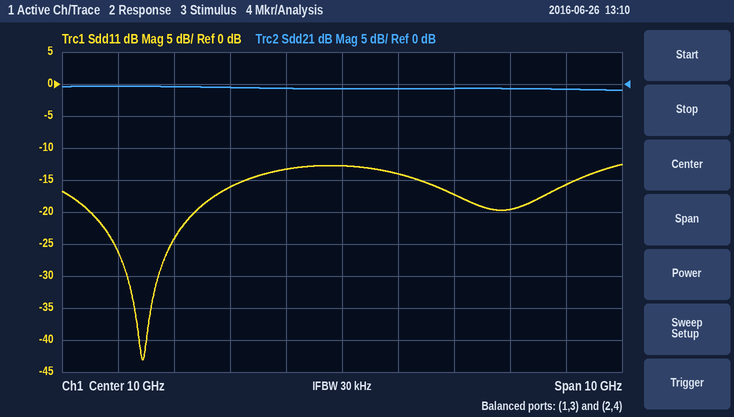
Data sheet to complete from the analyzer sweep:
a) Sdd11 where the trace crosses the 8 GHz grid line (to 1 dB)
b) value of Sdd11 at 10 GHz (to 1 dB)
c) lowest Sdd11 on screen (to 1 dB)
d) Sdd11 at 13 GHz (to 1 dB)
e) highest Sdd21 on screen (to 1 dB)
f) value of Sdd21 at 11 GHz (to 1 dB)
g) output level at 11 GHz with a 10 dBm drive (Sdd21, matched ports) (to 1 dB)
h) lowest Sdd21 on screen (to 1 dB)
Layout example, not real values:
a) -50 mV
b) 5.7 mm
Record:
a) -16 dB
b) -13 dB
c) -43 dB
d) -20 dB
e) 0 dB
f) -1 dB
g) 9 dBm
h) -1 dB
